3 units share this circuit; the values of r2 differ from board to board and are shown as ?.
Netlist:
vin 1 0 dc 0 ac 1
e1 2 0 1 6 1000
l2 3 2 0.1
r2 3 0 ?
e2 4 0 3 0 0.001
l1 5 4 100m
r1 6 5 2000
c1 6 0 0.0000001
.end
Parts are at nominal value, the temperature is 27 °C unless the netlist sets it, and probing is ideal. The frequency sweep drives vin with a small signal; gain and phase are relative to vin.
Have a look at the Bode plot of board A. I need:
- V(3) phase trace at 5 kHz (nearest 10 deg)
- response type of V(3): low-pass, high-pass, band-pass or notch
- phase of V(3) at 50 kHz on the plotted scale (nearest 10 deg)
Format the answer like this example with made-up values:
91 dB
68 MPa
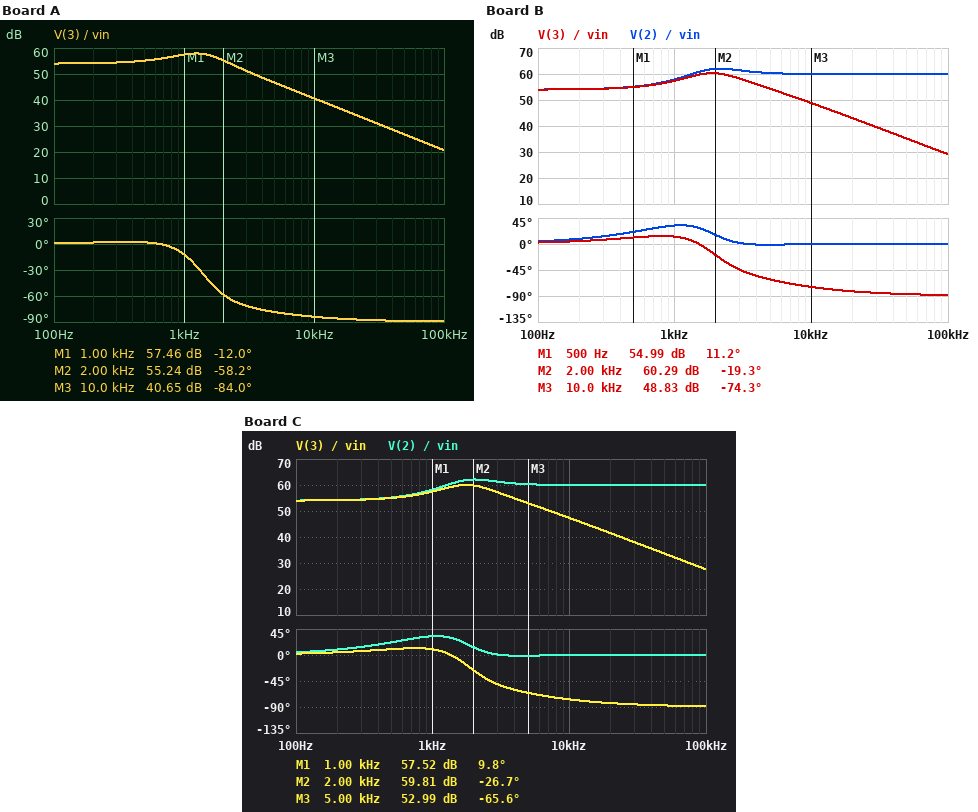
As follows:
-80 deg
low-pass
-90 deg
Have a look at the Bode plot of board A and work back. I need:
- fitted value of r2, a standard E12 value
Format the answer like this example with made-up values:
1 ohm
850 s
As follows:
680 Ω
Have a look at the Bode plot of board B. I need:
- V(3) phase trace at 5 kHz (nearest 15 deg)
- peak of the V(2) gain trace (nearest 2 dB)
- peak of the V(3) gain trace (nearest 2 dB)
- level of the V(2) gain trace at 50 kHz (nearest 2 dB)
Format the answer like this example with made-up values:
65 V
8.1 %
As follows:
-60 deg
62 dB
60 dB
60 dB
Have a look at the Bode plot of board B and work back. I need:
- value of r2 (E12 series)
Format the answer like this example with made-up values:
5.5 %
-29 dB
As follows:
1.8 kΩ
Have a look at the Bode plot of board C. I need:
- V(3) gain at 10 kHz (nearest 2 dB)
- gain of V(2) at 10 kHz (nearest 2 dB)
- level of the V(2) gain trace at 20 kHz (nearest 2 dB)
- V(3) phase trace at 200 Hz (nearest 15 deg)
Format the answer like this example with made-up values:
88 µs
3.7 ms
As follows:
48 dB
60 dB
60 dB
0 deg
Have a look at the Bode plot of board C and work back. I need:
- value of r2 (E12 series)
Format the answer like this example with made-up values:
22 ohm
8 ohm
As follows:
1.5 kΩ
